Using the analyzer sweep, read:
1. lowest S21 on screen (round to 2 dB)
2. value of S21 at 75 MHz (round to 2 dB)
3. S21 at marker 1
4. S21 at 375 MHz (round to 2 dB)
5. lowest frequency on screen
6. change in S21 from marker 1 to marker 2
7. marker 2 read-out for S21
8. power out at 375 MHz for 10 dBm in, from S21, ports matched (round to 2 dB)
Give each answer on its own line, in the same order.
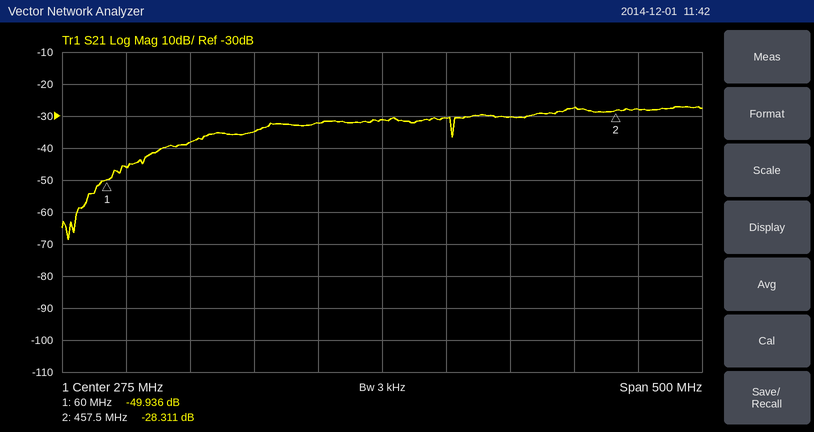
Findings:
-68 dB
-46 dB
-49.936 dB
-30 dB
25 MHz
21.625 dB
-28.311 dB
-20 dBm
